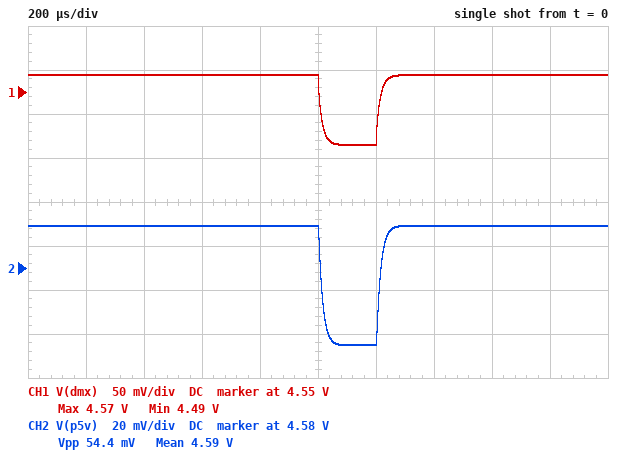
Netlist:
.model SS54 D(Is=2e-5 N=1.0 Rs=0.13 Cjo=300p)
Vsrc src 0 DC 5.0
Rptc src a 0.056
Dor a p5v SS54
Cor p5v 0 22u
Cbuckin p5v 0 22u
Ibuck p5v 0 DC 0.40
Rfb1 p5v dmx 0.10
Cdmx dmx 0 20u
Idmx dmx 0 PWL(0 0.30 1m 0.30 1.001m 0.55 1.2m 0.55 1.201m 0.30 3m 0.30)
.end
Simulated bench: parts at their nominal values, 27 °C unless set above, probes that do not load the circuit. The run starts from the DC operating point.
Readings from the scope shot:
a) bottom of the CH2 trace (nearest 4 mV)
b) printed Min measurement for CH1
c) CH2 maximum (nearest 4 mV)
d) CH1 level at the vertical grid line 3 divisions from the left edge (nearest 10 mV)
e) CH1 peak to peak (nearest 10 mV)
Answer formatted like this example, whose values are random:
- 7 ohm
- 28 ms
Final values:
- 4.544 V
- 4.49 V
- 4.600 V
- 4.57 V
- 80 mV
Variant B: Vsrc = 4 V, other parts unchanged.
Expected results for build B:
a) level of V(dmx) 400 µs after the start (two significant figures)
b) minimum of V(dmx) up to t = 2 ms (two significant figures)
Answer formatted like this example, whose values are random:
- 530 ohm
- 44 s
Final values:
- 3.6 V
- 3.5 V
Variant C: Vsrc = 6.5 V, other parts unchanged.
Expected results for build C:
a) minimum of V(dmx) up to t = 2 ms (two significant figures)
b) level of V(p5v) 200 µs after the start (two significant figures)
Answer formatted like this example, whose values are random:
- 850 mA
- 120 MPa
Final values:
- 6.0 V
- 6.1 V
